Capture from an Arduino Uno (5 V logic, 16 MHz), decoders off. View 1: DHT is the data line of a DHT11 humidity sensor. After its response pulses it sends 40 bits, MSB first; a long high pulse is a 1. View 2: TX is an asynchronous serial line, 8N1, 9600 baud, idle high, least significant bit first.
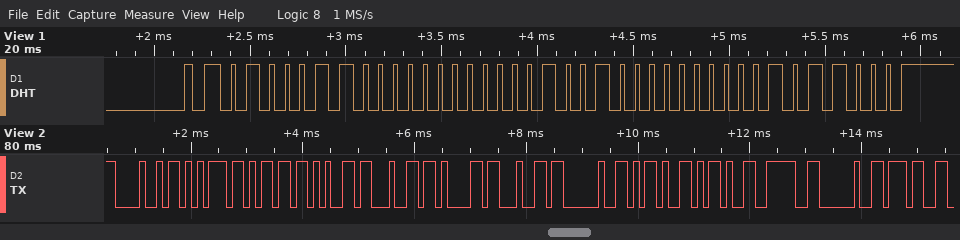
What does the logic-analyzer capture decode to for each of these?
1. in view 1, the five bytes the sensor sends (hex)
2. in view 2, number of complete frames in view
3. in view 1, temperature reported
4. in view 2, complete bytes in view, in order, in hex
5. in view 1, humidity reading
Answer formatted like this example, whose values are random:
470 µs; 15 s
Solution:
46 00 12 00 58; 13; 18.0 °C; 48 75 6D 65 64 61 64 20 2D 2D 3E 20 37; 70 %
